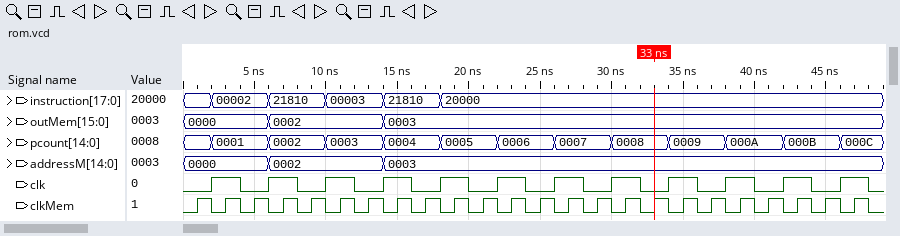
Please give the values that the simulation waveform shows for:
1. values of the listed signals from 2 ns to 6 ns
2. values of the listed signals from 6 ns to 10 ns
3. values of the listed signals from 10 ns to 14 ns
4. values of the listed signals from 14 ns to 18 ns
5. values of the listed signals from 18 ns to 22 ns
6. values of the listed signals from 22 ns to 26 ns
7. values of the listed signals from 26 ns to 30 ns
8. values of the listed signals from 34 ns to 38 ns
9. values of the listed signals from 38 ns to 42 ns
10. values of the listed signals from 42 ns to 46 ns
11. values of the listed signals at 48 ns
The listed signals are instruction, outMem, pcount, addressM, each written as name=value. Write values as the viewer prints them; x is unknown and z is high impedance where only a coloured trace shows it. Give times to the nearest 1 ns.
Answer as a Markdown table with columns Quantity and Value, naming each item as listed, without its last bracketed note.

| Quantity | Value |
|---|---|
| values of the listed signals from 2 ns to 6 ns | instruction=00002, outMem=0000, pcount=0001, addressM=0000 |
| values of the listed signals from 6 ns to 10 ns | instruction=21810, outMem=0002, pcount=0002, addressM=0002 |
| values of the listed signals from 10 ns to 14 ns | instruction=00003, outMem=0002, pcount=0003, addressM=0002 |
| values of the listed signals from 14 ns to 18 ns | instruction=21810, outMem=0003, pcount=0004, addressM=0003 |
| values of the listed signals from 18 ns to 22 ns | instruction=20000, outMem=0003, pcount=0005, addressM=0003 |
| values of the listed signals from 22 ns to 26 ns | instruction=20000, outMem=0003, pcount=0006, addressM=0003 |
| values of the listed signals from 26 ns to 30 ns | instruction=20000, outMem=0003, pcount=0007, addressM=0003 |
| values of the listed signals from 34 ns to 38 ns | instruction=20000, outMem=0003, pcount=0009, addressM=0003 |
| values of the listed signals from 38 ns to 42 ns | instruction=20000, outMem=0003, pcount=000A, addressM=0003 |
| values of the listed signals from 42 ns to 46 ns | instruction=20000, outMem=0003, pcount=000B, addressM=0003 |
| values of the listed signals at 48 ns | instruction=20000, outMem=0003, pcount=000C, addressM=0003 |
